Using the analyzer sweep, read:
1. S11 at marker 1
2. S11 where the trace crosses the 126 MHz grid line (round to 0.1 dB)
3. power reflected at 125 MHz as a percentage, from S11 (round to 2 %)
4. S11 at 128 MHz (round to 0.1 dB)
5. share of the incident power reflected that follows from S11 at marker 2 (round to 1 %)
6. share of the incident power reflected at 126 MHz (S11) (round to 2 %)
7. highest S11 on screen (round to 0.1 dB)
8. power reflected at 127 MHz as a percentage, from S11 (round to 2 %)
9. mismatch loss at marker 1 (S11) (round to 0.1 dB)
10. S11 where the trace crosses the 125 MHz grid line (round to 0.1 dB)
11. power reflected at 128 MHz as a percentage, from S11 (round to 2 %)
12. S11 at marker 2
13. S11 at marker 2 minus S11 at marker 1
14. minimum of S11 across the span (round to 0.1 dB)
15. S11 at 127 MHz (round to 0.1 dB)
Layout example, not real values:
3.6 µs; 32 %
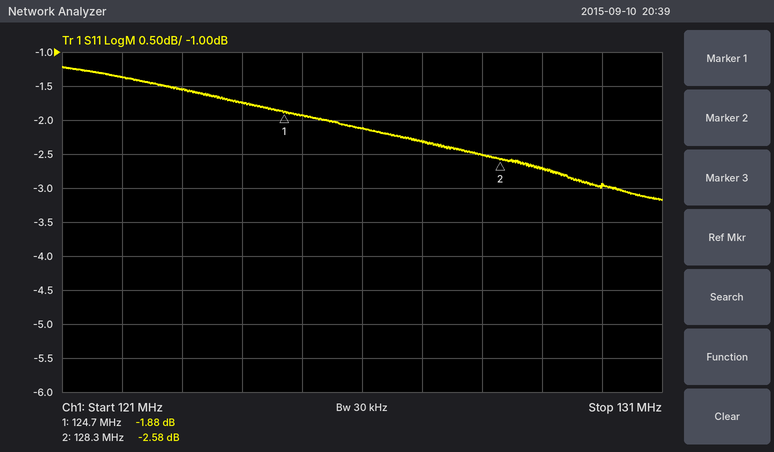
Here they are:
-1.88 dB; -2.1 dB; 64 %; -2.5 dB; 55 %; 62 %; -1.2 dB; 58 %; 4.5 dB; -1.9 dB; 56 %; -2.58 dB; -0.70 dB; -3.2 dB; -2.3 dB
